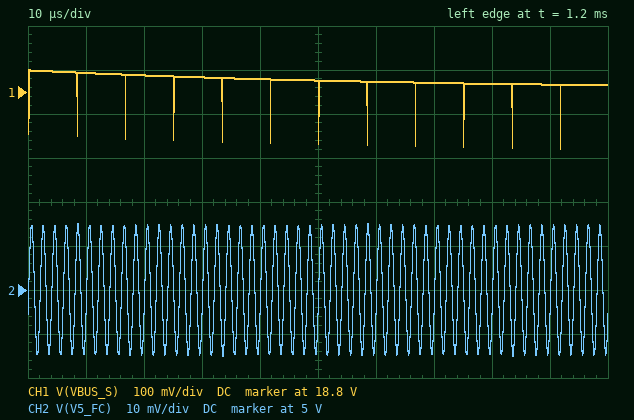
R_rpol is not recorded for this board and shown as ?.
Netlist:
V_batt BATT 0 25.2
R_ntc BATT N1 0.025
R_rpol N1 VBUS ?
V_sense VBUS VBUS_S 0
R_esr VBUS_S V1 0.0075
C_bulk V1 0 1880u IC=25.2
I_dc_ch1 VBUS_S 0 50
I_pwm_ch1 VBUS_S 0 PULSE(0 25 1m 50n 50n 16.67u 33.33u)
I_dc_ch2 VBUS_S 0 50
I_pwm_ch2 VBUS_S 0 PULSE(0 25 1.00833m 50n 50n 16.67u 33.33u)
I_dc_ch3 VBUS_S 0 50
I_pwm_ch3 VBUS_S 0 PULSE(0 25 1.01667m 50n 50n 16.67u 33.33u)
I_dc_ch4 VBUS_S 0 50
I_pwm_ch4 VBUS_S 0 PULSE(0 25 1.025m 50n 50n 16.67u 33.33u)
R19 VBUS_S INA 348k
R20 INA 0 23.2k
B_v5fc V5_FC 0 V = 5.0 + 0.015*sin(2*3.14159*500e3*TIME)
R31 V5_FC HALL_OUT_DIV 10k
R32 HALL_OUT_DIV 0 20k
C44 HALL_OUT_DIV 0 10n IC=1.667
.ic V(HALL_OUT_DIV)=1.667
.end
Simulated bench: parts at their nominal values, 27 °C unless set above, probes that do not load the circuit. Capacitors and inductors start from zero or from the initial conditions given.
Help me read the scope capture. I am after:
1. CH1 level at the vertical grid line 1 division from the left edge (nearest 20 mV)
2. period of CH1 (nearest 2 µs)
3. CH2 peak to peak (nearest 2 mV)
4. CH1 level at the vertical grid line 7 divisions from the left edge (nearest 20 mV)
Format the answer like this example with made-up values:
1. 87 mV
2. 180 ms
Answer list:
1. 18.84 V
2. 8 µs
3. 30 mV
4. 18.82 V
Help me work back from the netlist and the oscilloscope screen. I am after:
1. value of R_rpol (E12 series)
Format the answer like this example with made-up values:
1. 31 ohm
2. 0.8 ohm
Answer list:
1. 560 µΩ
